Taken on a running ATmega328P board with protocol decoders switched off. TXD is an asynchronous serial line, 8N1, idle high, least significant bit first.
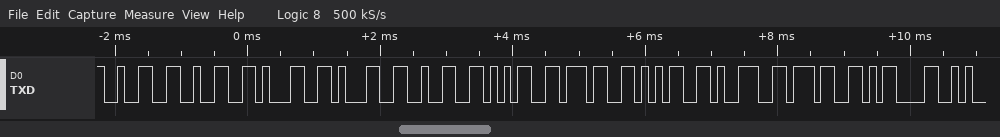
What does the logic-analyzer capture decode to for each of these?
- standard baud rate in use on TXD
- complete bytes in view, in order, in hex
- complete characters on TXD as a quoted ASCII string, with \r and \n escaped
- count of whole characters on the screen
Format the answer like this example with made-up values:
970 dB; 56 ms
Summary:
9600 baud; 0x32 0x32 0x31 0x31 0x32 0x35 0x37 0x35 0x39 0x37 0x0D; "2211257597\r"; 11
